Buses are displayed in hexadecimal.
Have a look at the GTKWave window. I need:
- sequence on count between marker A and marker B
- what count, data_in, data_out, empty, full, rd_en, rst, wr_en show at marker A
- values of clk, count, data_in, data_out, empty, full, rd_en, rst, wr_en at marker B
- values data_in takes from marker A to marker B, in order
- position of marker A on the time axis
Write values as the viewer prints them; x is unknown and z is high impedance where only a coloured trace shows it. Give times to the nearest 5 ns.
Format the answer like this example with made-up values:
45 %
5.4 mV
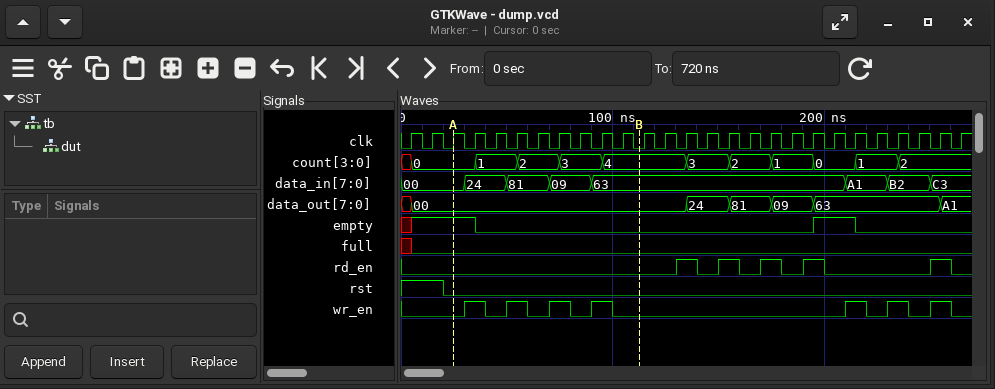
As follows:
0, 1, 2, 3, 4
count=0, data_in=00, data_out=00, empty=1, full=0, rd_en=0, rst=0, wr_en=0
clk=0, count=4, data_in=63, data_out=00, empty=0, full=0, rd_en=0, rst=0, wr_en=0
00, 24, 81, 09, 63
25 ns
